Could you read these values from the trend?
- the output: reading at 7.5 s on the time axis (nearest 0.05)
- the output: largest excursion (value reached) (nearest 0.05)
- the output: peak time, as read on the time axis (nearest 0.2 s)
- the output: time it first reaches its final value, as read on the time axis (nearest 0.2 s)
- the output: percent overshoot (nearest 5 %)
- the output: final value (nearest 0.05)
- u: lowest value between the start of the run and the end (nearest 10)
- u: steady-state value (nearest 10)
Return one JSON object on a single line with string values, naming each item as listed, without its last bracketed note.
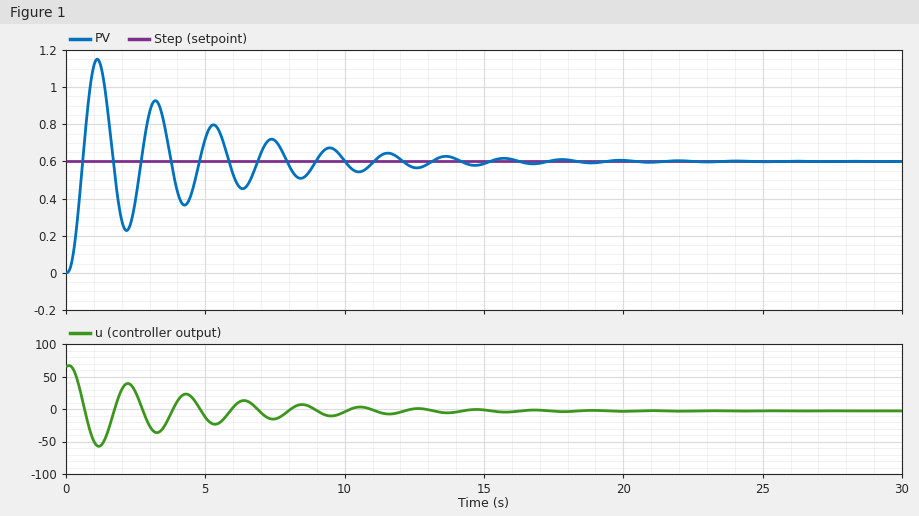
{"the output: reading at 7.5 s on the time axis": "0.70", "the output: largest excursion (value reached)": "1.15", "the output: peak time, as read on the time axis": "1.2 s", "the output: time it first reaches its final value, as read on the time axis": "0.6 s", "the output: percent overshoot": "90 %", "the output: final value": "0.60", "u: lowest value between the start of the run and the end": "-60", "u: steady-state value": "0"}
